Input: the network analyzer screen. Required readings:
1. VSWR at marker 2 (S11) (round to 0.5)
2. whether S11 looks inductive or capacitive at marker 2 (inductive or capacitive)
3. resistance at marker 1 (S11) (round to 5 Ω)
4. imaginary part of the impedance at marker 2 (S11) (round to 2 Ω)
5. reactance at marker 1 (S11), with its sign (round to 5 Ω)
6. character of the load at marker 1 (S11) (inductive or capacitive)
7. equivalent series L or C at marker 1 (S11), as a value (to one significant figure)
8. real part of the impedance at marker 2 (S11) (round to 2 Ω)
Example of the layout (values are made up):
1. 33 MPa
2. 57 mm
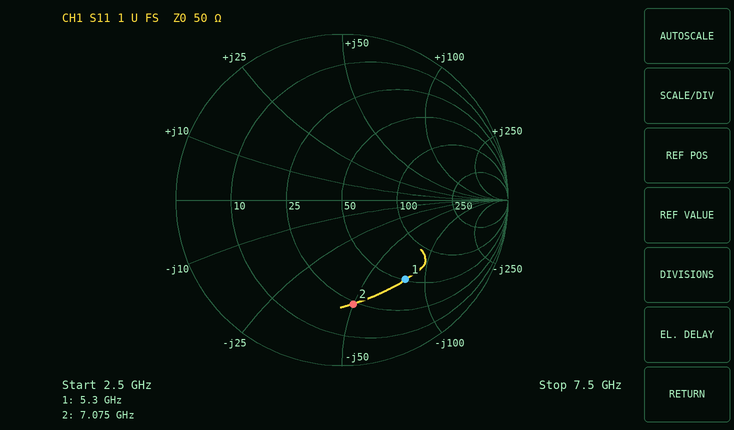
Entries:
1. 4.5
2. capacitive
3. 50 Ω
4. -50 Ω
5. -80 Ω
6. capacitive
7. 400 fF
8. 24 Ω
